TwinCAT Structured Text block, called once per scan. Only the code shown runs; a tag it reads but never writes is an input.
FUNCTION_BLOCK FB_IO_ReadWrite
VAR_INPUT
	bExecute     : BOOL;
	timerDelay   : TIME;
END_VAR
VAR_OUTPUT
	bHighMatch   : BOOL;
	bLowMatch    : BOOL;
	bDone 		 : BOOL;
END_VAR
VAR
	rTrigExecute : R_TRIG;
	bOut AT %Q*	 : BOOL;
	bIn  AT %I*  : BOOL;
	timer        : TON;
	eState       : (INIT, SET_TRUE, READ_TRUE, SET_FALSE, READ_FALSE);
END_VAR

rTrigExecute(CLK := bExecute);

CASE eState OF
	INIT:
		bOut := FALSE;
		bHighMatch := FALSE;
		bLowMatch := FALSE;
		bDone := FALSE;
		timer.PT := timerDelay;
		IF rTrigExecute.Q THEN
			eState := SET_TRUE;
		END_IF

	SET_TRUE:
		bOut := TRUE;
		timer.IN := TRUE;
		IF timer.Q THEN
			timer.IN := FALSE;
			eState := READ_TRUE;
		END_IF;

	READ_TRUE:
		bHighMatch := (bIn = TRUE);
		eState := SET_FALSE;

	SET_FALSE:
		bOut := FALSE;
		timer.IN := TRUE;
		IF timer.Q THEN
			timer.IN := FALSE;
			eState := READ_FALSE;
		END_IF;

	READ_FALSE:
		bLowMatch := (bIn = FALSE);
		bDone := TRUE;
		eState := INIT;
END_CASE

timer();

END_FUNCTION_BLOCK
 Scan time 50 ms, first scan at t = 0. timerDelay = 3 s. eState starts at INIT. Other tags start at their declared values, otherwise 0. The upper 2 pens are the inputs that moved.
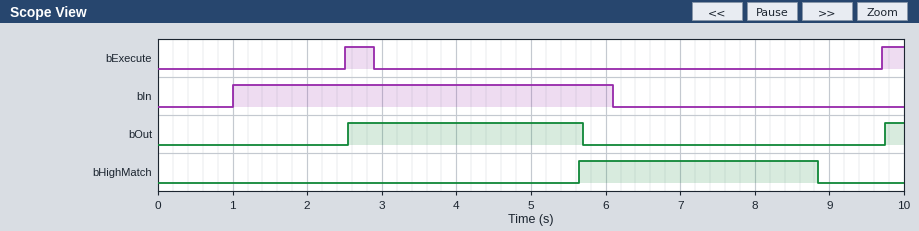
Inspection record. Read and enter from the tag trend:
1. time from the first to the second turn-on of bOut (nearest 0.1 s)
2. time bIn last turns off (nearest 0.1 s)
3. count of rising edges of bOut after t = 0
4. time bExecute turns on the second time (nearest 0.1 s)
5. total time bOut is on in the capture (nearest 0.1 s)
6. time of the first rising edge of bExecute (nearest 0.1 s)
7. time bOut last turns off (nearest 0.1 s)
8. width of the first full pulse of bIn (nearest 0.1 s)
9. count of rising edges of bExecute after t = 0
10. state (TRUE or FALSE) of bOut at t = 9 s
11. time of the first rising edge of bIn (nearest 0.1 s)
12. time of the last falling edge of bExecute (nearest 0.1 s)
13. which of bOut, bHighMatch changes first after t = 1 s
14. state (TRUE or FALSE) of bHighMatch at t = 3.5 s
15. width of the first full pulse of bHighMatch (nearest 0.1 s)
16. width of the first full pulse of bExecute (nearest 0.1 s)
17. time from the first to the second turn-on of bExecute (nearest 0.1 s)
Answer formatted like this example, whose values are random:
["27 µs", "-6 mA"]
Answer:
["7.2 s", "6.1 s", "2", "9.7 s", "3.4 s", "2.5 s", "5.7 s", "5.1 s", "2", "FALSE", "1.0 s", "2.9 s", "bOut", "FALSE", "3.2 s", "0.4 s", "7.2 s"]
